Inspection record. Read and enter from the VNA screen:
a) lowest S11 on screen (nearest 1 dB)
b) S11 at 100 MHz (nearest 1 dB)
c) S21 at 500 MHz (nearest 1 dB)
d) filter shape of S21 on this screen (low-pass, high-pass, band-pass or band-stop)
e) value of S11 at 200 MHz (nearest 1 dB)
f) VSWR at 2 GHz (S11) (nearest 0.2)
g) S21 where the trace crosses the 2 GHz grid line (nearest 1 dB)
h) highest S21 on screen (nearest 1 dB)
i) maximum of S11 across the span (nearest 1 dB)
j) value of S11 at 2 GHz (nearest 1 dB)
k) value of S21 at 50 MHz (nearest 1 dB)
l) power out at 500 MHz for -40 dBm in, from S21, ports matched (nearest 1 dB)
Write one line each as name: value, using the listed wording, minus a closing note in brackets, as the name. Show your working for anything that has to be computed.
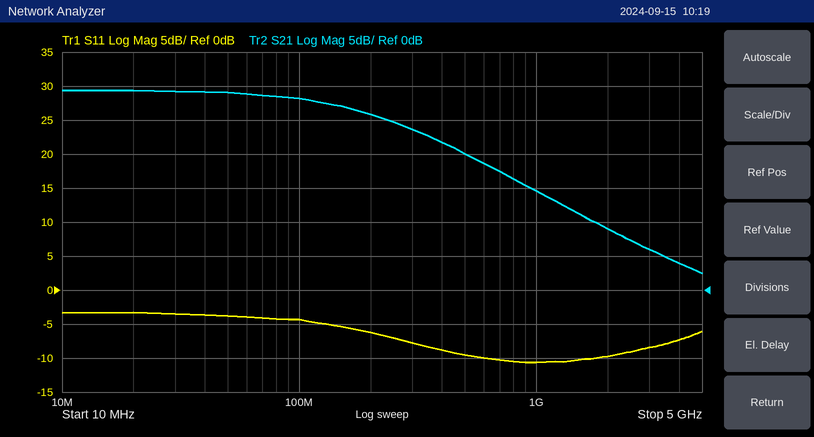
lowest S11 on screen: -11 dB
S11 at 100 MHz: -4 dB
S21 at 500 MHz: 20 dB
filter shape of S21 on this screen: low-pass
value of S11 at 200 MHz: -6 dB
VSWR at 2 GHz (S11): |Γ| = 10^(-10/20) = 0.3162; VSWR = (1 + 0.3162)/(1 − 0.3162) ≈ 1.92, so 2.0 to the nearest 0.2
S21 where the trace crosses the 2 GHz grid line: 9 dB
highest S21 on screen: 29 dB
maximum of S11 across the span: -3 dB
value of S11 at 2 GHz: -10 dB
value of S21 at 50 MHz: 29 dB
power out at 500 MHz for -40 dBm in, from S21, ports matched: -40 dBm + (20 dB) = -20 dBm
